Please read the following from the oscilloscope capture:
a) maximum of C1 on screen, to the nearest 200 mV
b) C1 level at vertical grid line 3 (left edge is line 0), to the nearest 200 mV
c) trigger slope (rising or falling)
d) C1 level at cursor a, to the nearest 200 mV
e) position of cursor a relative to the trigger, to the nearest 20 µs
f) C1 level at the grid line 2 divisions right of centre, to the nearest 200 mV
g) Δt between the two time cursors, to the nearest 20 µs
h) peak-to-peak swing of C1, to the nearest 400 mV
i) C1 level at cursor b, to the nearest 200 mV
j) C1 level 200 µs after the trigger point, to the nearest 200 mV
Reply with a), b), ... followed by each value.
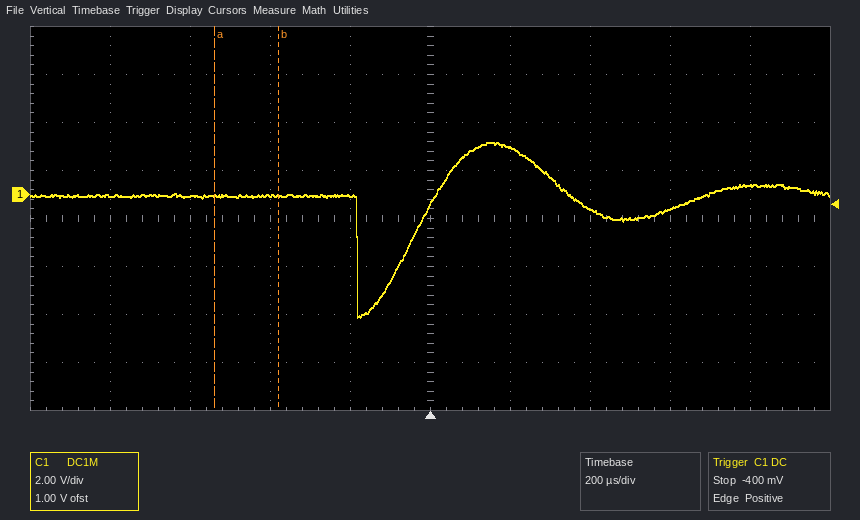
a) 2.2 V
b) 0.0 V
c) rising
d) 0.0 V
e) -540 µs
f) -600 mV
g) 160 µs
h) 7.2 V
i) 0.0 V
j) 2.0 V
